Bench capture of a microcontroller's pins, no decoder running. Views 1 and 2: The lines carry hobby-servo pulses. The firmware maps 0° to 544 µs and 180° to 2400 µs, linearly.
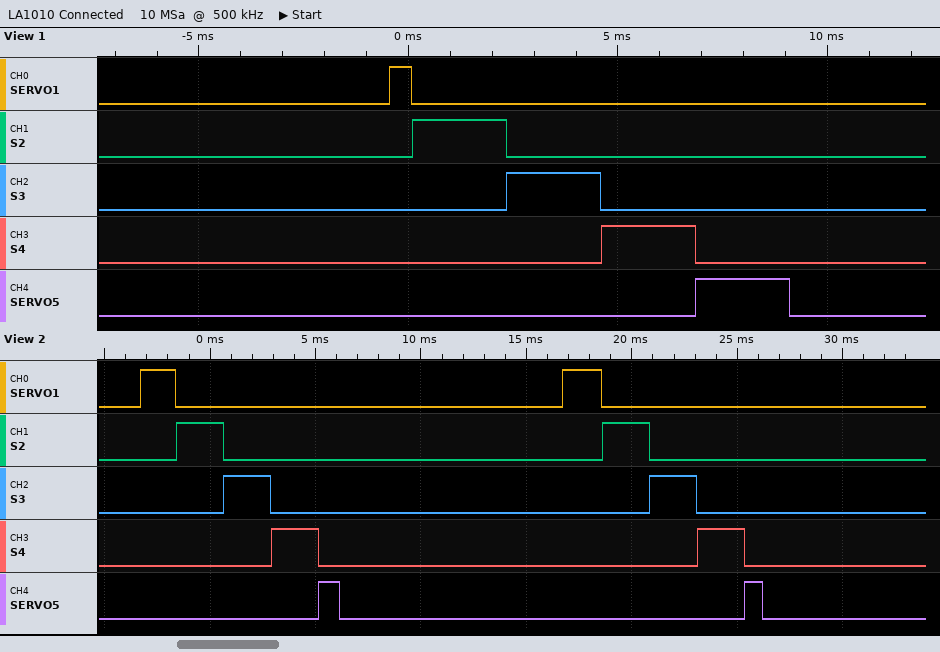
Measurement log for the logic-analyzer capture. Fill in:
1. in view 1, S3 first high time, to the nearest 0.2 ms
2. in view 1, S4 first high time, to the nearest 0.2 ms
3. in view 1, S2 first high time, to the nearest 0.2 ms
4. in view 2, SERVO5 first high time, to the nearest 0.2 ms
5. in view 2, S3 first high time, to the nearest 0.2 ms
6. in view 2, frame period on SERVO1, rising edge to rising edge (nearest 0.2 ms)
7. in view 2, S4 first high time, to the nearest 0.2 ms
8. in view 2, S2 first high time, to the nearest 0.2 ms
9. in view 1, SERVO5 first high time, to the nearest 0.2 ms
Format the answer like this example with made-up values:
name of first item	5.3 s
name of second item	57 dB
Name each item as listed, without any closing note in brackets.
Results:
in view 1, S3 first high time, to the nearest 0.2 ms	2.2 ms
in view 1, S4 first high time, to the nearest 0.2 ms	2.2 ms
in view 1, S2 first high time, to the nearest 0.2 ms	2.2 ms
in view 2, SERVO5 first high time, to the nearest 0.2 ms	1.0 ms
in view 2, S3 first high time, to the nearest 0.2 ms	2.2 ms
in view 2, frame period on SERVO1, rising edge to rising edge	20.0 ms
in view 2, S4 first high time, to the nearest 0.2 ms	2.2 ms
in view 2, S2 first high time, to the nearest 0.2 ms	2.2 ms
in view 1, SERVO5 first high time, to the nearest 0.2 ms	2.2 ms
